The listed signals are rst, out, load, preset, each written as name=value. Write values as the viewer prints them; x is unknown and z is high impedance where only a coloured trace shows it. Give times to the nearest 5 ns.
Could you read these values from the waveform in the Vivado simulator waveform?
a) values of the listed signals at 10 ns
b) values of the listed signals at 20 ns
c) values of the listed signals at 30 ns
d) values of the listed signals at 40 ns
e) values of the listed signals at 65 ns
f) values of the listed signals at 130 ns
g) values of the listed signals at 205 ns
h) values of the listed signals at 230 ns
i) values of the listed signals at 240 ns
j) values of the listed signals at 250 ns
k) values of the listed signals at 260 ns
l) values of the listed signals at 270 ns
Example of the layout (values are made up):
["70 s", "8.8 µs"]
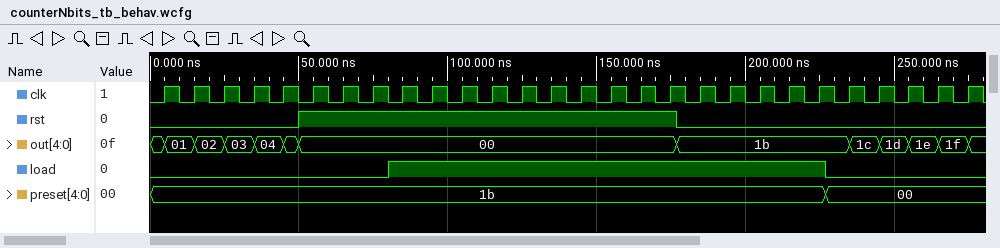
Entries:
["rst=0, out=01, load=0, preset=1b", "rst=0, out=02, load=0, preset=1b", "rst=0, out=03, load=0, preset=1b", "rst=0, out=04, load=0, preset=1b", "rst=1, out=00, load=0, preset=1b", "rst=1, out=00, load=1, preset=1b", "rst=0, out=1b, load=1, preset=1b", "rst=0, out=1b, load=0, preset=00", "rst=0, out=1c, load=0, preset=00", "rst=0, out=1d, load=0, preset=00", "rst=0, out=1e, load=0, preset=00", "rst=0, out=1f, load=0, preset=00"]
